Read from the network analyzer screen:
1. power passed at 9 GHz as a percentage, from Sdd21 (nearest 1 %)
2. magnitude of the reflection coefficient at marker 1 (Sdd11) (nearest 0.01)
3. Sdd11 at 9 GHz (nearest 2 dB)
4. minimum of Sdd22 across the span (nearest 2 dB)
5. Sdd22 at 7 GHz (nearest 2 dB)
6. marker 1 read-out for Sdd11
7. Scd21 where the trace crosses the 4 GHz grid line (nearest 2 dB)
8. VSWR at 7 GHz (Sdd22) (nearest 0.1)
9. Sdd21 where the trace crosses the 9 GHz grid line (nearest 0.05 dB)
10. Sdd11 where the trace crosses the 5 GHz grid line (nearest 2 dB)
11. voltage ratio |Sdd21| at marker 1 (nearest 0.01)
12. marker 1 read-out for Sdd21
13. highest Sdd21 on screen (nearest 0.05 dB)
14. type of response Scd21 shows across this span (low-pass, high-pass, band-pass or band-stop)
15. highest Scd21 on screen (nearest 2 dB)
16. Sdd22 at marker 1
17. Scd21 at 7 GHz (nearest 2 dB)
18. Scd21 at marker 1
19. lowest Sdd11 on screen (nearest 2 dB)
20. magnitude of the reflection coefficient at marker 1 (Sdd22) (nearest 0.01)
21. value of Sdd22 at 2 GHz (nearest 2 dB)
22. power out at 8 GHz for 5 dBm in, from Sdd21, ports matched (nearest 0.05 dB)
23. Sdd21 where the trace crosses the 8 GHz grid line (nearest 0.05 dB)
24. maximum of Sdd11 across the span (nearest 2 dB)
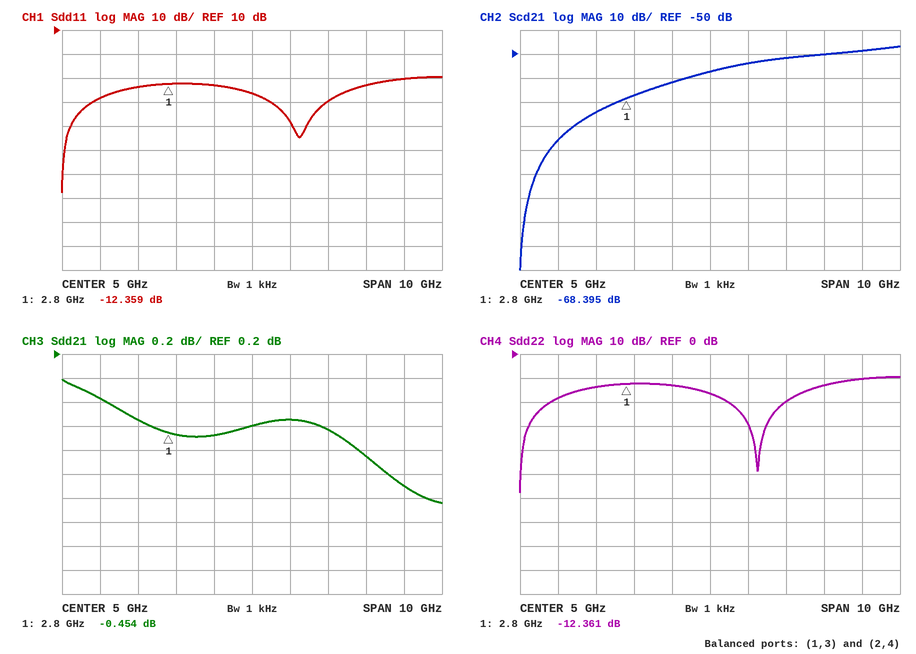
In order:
81 %
0.24
-10 dB
-58 dB
-20 dB
-12.359 dB
-62 dB
1.2
-0.90 dB
-16 dB
0.95
-0.454 dB
0.00 dB
high-pass
-46 dB
-12.361 dB
-52 dB
-68.395 dB
-58 dB
0.24
-14 dB
4.35 dBm
-0.65 dB
-10 dB
